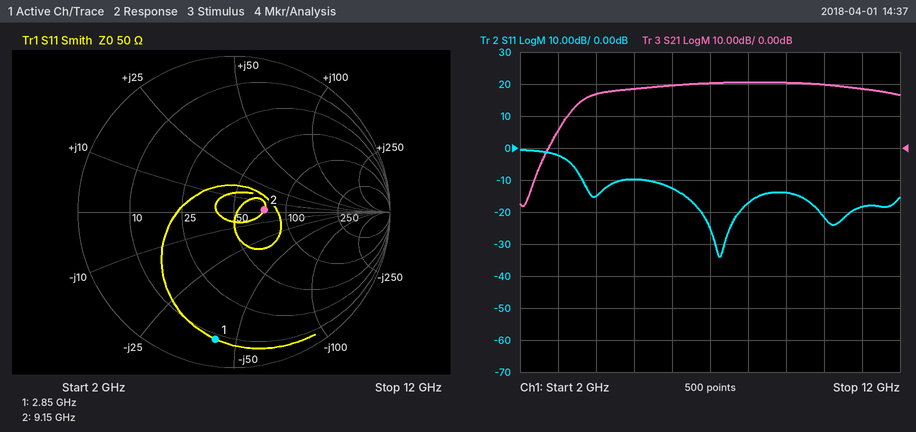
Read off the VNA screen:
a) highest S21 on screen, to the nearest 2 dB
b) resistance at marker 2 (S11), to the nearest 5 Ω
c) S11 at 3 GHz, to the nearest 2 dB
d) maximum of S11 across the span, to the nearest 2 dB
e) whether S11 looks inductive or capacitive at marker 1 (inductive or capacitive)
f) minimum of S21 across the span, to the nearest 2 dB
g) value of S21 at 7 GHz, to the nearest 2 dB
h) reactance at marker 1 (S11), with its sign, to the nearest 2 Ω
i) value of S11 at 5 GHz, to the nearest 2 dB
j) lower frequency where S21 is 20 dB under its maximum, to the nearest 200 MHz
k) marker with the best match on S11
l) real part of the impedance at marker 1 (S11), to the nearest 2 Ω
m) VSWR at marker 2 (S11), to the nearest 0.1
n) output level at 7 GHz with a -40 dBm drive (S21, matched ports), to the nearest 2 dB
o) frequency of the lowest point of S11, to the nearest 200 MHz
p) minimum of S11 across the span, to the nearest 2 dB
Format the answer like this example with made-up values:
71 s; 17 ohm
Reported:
20 dB; 75 Ω; -2 dB; 0 dB; capacitive; -18 dB; 20 dB; -42 Ω; -10 dB; 2.8 GHz; marker 2; 8 Ω; 1.5; -20 dBm; 7.2 GHz; -34 dB
